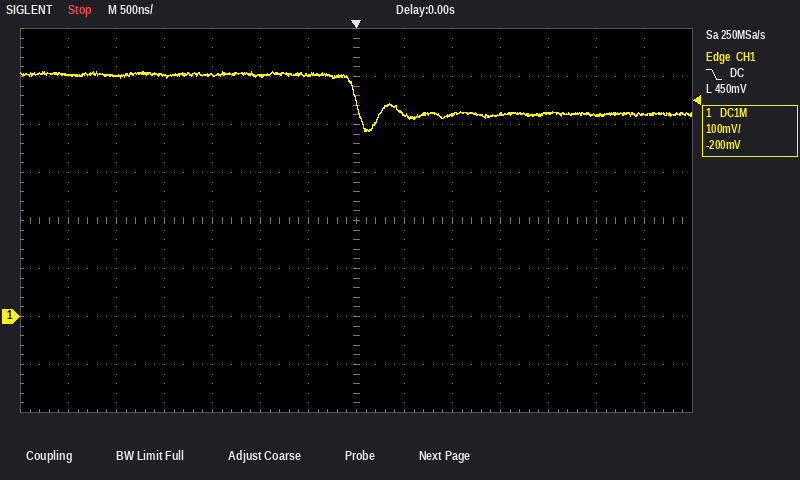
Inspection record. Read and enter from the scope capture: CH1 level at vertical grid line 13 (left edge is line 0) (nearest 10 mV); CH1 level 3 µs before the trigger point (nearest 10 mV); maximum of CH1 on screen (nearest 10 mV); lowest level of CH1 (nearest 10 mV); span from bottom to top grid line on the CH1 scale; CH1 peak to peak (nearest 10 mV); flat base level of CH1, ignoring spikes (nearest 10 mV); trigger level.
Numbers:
420 mV
500 mV
510 mV
390 mV
800 mV
120 mV
420 mV
450 mV
